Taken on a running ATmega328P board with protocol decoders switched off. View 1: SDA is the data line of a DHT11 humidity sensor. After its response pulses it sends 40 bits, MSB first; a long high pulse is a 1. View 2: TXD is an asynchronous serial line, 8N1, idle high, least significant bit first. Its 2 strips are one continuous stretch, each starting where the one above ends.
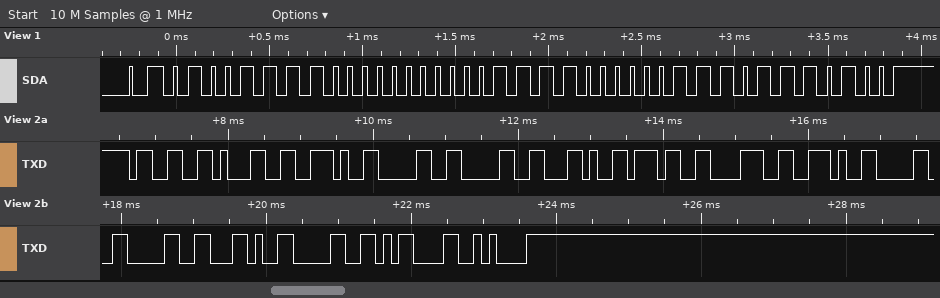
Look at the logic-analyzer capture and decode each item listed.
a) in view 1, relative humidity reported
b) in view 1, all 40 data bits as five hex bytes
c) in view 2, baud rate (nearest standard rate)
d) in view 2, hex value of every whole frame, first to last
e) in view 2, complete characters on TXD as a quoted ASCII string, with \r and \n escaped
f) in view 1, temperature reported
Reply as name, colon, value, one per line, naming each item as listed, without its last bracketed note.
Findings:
in view 1, relative humidity reported: 79 %
in view 1, all 40 data bits as five hex bytes: 4F 00 1E 07 74
in view 2, baud rate: 9600 baud
in view 2, hex value of every whole frame, first to last: 33 31 2E 30 30 2C 37 38 2E 30 30 2C 30 0D 0A
in view 2, complete characters on TXD as a quoted ASCII string, with \r and \n escaped: "31.00,78.00,0\r\n"
in view 1, temperature reported: 30.7 °C
